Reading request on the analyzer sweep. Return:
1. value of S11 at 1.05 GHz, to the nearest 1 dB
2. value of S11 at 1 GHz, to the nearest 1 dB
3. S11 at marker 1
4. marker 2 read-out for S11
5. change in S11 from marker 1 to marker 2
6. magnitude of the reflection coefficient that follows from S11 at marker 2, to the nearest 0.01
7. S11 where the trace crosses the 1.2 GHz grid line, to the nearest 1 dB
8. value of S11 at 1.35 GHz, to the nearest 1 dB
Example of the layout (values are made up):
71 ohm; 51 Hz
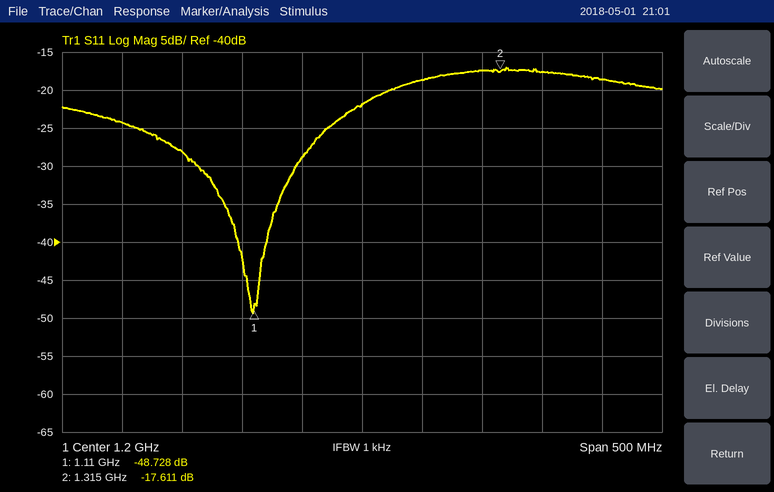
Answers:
-28 dB; -24 dB; -48.728 dB; -17.611 dB; 31.117 dB; 0.13; -22 dB; -18 dB
